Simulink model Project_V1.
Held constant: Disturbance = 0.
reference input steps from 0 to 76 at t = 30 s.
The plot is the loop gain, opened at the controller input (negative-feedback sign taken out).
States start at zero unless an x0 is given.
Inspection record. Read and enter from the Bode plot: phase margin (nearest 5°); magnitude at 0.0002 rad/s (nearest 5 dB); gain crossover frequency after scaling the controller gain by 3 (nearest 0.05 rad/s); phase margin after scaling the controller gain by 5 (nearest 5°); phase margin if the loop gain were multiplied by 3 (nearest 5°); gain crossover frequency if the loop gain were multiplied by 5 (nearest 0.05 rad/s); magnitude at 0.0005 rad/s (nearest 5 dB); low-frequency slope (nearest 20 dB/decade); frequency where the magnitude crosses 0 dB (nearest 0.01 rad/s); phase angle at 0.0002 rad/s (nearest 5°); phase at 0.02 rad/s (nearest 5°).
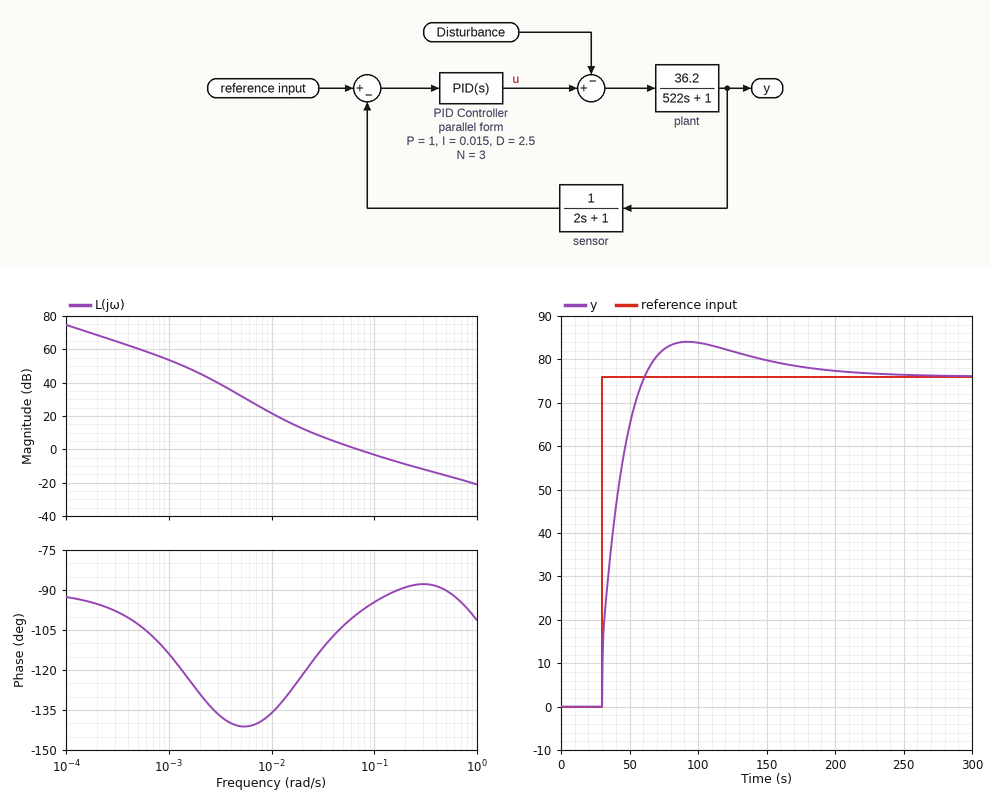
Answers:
80°
70 dB
0.20 rad/s
90°
90°
0.40 rad/s
60 dB
-20 dB/decade
0.07 rad/s
-95°
-120°
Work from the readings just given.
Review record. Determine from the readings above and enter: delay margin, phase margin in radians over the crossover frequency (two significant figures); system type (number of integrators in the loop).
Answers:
20 s
1
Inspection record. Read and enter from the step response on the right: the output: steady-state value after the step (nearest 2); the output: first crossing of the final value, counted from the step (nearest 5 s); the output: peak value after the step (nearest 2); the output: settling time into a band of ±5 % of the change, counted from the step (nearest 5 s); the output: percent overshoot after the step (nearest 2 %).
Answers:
76
30 s
84
120 s
10 %
